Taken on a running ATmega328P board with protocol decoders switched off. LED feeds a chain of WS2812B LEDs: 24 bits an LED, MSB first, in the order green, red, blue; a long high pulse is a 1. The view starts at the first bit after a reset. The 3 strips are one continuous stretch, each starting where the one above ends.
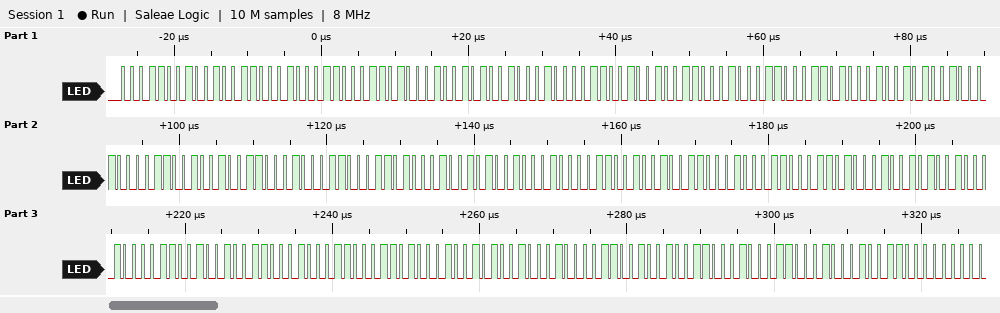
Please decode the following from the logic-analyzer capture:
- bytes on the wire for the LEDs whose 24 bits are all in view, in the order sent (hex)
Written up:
19 26 23 1A 25 22 19 26 23 1A 25 22 19 26 23 1A 25 22 19 26 23 1A 25 22 19 26 23 1A 25 22 19 26 23
